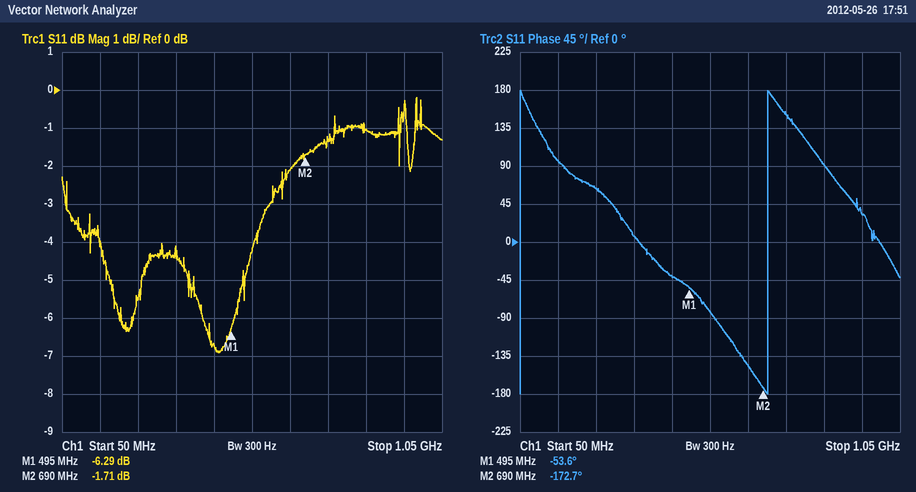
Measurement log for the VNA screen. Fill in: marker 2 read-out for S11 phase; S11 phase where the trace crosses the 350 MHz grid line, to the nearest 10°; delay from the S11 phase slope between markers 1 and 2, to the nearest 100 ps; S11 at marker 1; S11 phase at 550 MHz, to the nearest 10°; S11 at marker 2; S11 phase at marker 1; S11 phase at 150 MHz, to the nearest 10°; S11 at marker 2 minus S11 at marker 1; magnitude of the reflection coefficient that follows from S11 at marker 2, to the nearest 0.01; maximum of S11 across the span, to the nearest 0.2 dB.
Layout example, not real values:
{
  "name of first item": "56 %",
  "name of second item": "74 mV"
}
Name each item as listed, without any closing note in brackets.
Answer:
{
  "marker 2 read-out for S11 phase": "-172.7°",
  "S11 phase where the trace crosses the 350 MHz grid line, to the nearest 10°": "10°",
  "delay from the S11 phase slope between markers 1 and 2, to the nearest 100 ps": "1.7 ns",
  "S11 at marker 1": "-6.29 dB",
  "S11 phase at 550 MHz, to the nearest 10°": "-80°",
  "S11 at marker 2": "-1.71 dB",
  "S11 phase at marker 1": "-53.6°",
  "S11 phase at 150 MHz, to the nearest 10°": "100°",
  "S11 at marker 2 minus S11 at marker 1": "4.58 dB",
  "magnitude of the reflection coefficient that follows from S11 at marker 2, to the nearest 0.01": "0.82",
  "maximum of S11 across the span, to the nearest 0.2 dB": "-0.2 dB"
}
